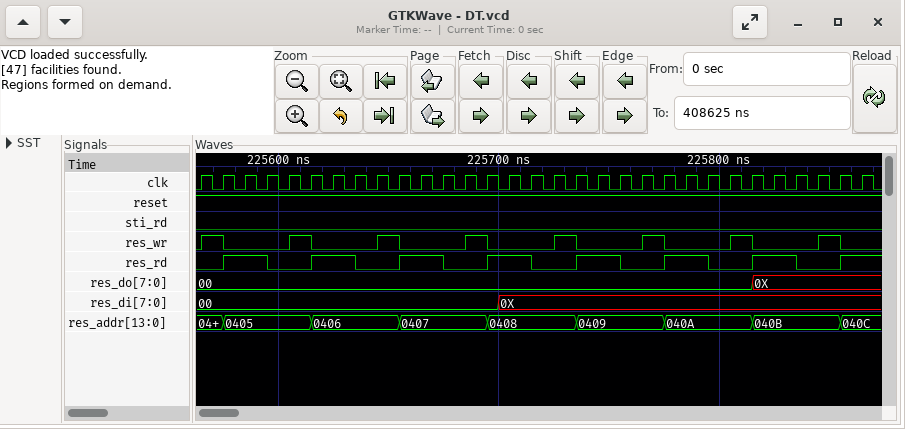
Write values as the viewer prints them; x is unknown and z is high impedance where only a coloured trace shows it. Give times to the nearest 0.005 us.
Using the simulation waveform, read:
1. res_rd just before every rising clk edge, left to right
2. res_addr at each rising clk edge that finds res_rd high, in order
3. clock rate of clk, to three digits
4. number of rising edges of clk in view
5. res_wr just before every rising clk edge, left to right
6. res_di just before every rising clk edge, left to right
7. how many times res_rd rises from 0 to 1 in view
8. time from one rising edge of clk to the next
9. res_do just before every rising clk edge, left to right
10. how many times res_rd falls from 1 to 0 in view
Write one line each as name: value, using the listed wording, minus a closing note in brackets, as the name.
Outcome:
res_rd just before every rising clk edge, left to right: 0 0 1 1 0 0 1 1 0 0 1 1 0 0 1 1 0 0 1 1 0 0 1 1 0 0 1 1 0 0 1
res_addr at each rising clk edge that finds res_rd high, in order: 0405, 0405, 0406, 0406, 0407, 0407, 0408, 0408, 0409, 0409, 040A, 040A, 040B, 040B, 040C
clock rate of clk, to three digits: 100 MHz
number of rising edges of clk in view: 31
res_wr just before every rising clk edge, left to right: 0 1 0 0 0 1 0 0 0 1 0 0 0 1 0 0 0 1 0 0 0 1 0 0 0 1 0 0 0 1 0
res_di just before every rising clk edge, left to right: 00, 00, 00, 00, 00, 00, 00, 00, 00, 00, 00, 00, 00, 00, 0X, 0X, 0X, 0X, 0X, 0X, 0X, 0X, 0X, 0X, 0X, 0X, 0X, 0X, 0X, 0X, 0X
how many times res_rd rises from 0 to 1 in view: 8
time from one rising edge of clk to the next: 0.01 us
res_do just before every rising clk edge, left to right: 00, 00, 00, 00, 00, 00, 00, 00, 00, 00, 00, 00, 00, 00, 00, 00, 00, 00, 00, 00, 00, 00, 00, 00, 00, 00, 0X, 0X, 0X, 0X, 0X
how many times res_rd falls from 1 to 0 in view: 7
